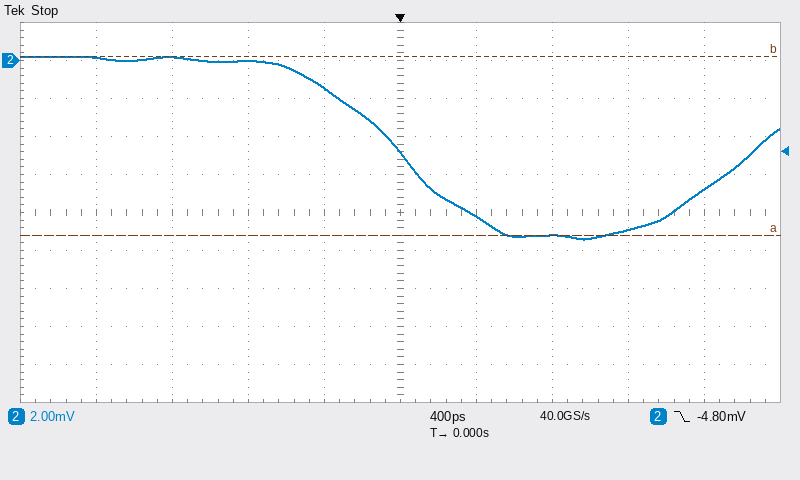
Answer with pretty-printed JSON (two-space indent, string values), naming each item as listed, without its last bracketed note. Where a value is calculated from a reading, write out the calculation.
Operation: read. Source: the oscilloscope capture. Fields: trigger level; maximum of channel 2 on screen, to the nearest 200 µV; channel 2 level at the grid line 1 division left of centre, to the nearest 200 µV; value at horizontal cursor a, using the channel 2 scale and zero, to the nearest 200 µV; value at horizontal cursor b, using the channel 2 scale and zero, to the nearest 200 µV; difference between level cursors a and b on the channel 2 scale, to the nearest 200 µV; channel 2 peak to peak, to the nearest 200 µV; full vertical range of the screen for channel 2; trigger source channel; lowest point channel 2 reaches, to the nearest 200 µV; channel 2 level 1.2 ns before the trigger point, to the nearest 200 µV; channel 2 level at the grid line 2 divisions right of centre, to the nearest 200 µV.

{
  "trigger level": "-4.80 mV",
  "maximum of channel 2 on screen, to the nearest 200 µV": "200 µV",
  "channel 2 level at the grid line 1 division left of centre, to the nearest 200 µV": "-1.4 mV",
  "value at horizontal cursor a, using the channel 2 scale and zero, to the nearest 200 µV": "-9.2 mV",
  "value at horizontal cursor b, using the channel 2 scale and zero, to the nearest 200 µV": "200 µV",
  "difference between level cursors a and b on the channel 2 scale, to the nearest 200 µV": "9.4 mV",
  "channel 2 peak to peak, to the nearest 200 µV": "200 µV − (-9.4 mV) = 9.6 mV",
  "full vertical range of the screen for channel 2": "20 mV",
  "trigger source channel": "channel 2",
  "lowest point channel 2 reaches, to the nearest 200 µV": "-9.4 mV",
  "channel 2 level 1.2 ns before the trigger point, to the nearest 200 µV": "200 µV",
  "channel 2 level at the grid line 2 divisions right of centre, to the nearest 200 µV": "-9.2 mV"
}
